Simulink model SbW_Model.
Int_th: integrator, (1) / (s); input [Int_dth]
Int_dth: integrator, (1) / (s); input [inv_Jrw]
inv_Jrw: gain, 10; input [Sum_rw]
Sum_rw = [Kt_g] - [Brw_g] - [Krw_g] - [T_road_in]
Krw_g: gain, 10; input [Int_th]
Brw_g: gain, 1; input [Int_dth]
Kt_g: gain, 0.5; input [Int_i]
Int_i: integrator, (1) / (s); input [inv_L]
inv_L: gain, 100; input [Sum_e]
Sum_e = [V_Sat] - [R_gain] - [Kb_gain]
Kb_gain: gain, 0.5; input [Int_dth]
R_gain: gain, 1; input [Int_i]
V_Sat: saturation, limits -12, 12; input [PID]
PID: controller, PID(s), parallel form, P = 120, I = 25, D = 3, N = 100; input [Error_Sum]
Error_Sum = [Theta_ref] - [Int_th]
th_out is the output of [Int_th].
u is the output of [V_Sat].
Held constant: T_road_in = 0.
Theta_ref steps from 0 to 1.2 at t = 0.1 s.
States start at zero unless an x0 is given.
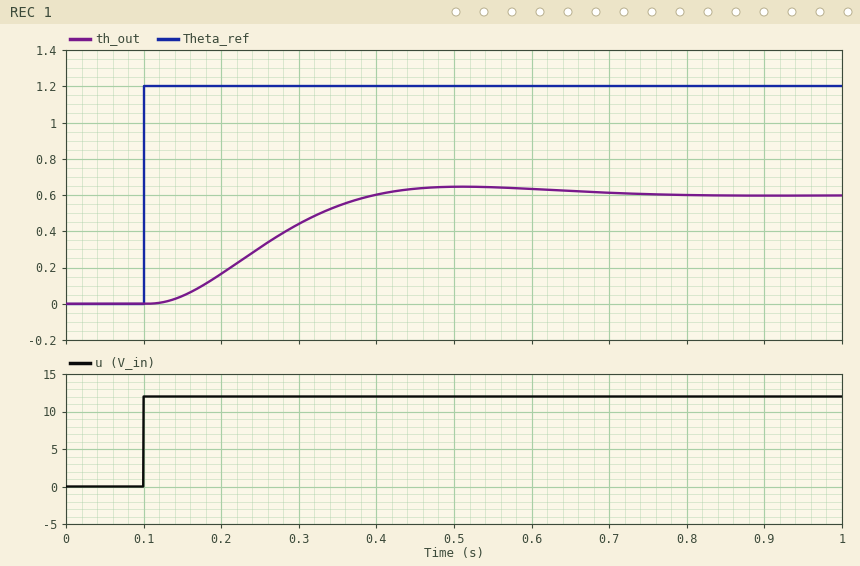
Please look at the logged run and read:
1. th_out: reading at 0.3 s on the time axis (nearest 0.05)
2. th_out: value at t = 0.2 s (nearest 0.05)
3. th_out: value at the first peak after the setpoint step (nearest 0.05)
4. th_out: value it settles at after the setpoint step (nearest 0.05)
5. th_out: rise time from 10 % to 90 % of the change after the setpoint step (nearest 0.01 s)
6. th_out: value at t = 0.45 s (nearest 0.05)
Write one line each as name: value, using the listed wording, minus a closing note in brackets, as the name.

th_out: reading at 0.3 s on the time axis: 0.45
th_out: value at t = 0.2 s: 0.15
th_out: value at the first peak after the setpoint step: 0.65
th_out: value it settles at after the setpoint step: 0.60
th_out: rise time from 10 % to 90 % of the change after the setpoint step: 0.19 s
th_out: value at t = 0.45 s: 0.65
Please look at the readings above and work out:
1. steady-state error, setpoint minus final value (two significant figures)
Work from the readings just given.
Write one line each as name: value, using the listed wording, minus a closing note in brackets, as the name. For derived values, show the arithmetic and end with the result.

steady-state error, setpoint minus final value: 1.2 - 0.6 = 0.60
